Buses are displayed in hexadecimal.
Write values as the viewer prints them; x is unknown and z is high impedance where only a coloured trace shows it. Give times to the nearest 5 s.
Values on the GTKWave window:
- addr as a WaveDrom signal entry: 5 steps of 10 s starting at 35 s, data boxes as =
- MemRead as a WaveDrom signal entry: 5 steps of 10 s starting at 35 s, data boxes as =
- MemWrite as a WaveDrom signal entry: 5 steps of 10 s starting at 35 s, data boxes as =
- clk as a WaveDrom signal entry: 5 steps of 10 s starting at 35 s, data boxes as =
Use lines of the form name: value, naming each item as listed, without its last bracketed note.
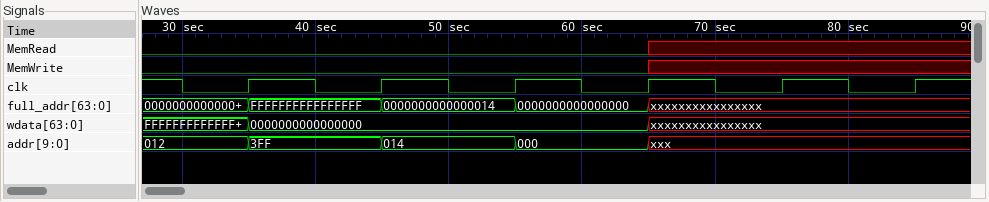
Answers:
addr as a WaveDrom signal entry: 5 steps of 10 s starting at 35 s, data boxes as =: {name: 'addr', wave: '===x.', data: '3FF 014 000'}
MemRead as a WaveDrom signal entry: 5 steps of 10 s starting at 35 s, data boxes as =: {name: 'MemRead', wave: '0..x.'}
MemWrite as a WaveDrom signal entry: 5 steps of 10 s starting at 35 s, data boxes as =: {name: 'MemWrite', wave: '0..x.'}
clk as a WaveDrom signal entry: 5 steps of 10 s starting at 35 s, data boxes as =: {name: 'clk', wave: 'p....'}
